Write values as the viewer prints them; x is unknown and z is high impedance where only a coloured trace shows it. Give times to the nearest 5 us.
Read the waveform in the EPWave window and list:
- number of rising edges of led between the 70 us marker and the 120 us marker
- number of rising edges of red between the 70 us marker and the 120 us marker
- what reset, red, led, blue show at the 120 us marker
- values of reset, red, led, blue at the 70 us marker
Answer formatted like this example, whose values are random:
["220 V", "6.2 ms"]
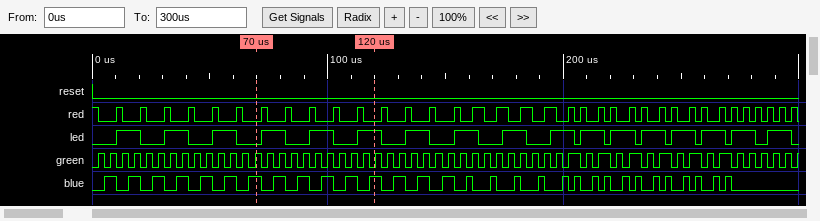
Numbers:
["3", "5", "reset=0, red=0, led=1, blue=1", "reset=0, red=0, led=0, blue=1"]
